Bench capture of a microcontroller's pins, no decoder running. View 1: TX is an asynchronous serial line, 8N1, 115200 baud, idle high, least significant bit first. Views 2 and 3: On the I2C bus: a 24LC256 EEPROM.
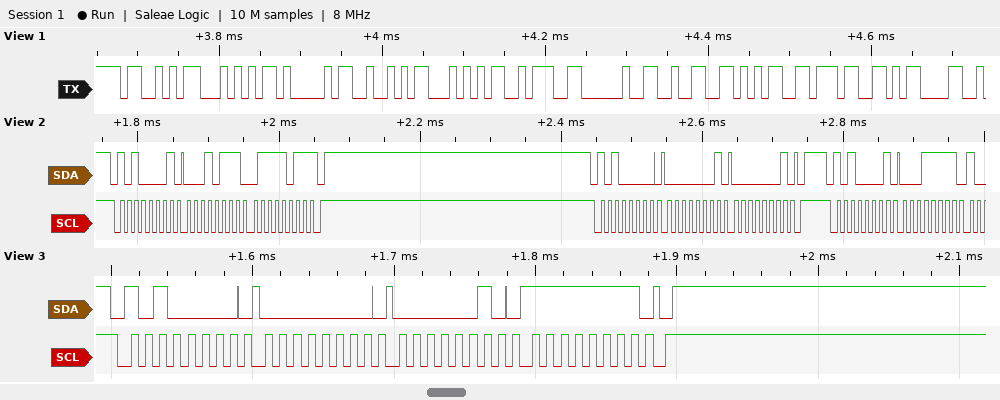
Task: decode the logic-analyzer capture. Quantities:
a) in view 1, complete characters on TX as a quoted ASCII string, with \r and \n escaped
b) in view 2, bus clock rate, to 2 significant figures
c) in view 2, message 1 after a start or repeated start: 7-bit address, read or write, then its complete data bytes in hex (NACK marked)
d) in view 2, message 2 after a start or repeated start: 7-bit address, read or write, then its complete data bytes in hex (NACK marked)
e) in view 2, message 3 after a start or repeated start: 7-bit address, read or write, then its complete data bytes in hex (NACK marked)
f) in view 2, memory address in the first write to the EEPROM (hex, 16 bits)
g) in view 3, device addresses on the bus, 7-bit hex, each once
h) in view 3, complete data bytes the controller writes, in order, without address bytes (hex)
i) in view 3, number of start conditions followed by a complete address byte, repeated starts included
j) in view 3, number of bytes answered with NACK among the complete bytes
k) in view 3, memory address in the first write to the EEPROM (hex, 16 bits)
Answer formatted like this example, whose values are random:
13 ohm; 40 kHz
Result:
"START: 257\r"; 100 kHz; 0x50 read: 17 7B NACK; 0x50 write: 01 01; 0x50 read: 1F; 0x0101; 0x50; 00 02 FF; 1; 0; 0x0002
